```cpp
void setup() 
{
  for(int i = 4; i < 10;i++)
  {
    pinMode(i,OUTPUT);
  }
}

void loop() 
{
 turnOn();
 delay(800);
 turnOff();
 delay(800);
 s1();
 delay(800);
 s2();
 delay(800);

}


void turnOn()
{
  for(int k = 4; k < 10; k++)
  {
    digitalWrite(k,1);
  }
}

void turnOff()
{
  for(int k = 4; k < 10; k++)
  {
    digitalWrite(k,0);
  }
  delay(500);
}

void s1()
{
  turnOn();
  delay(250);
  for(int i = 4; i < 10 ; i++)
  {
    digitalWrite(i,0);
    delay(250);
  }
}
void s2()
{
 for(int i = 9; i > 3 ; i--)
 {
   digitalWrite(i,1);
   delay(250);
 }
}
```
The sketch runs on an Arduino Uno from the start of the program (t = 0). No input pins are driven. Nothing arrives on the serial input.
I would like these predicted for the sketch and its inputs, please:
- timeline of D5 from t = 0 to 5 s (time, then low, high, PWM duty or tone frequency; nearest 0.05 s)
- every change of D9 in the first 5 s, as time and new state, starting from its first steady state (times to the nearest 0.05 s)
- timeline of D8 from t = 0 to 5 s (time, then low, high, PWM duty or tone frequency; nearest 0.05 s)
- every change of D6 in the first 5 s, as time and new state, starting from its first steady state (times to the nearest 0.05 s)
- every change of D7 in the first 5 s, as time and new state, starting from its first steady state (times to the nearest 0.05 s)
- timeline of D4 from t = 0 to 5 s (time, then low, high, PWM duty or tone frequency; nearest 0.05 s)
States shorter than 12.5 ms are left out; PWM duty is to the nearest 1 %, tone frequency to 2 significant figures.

0 s high; 0.8 s low; 2.1 s high; 2.6 s low
0 s high; 0.8 s low; 2.1 s high; 3.6 s low; 4.65 s high
0 s high; 0.8 s low; 2.1 s high; 3.35 s low; 4.9 s high
0 s high; 0.8 s low; 2.1 s high; 2.85 s low
0 s high; 0.8 s low; 2.1 s high; 3.1 s low
0 s high; 0.8 s low; 2.1 s high; 2.35 s low
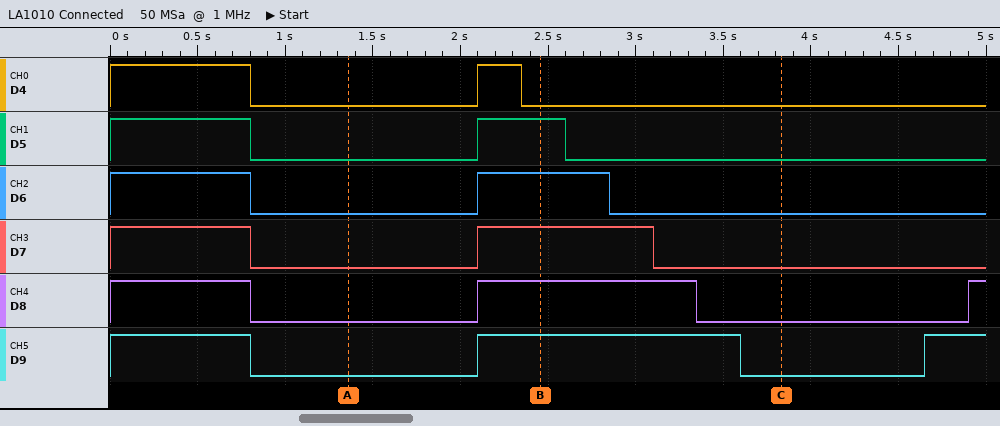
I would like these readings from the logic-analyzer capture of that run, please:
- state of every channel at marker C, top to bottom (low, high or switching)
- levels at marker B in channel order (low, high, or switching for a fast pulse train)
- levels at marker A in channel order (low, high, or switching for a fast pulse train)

D4 low, D5 low, D6 low, D7 low, D8 low, D9 low
D4 low, D5 high, D6 high, D7 high, D8 high, D9 high
D4 low, D5 low, D6 low, D7 low, D8 low, D9 low
